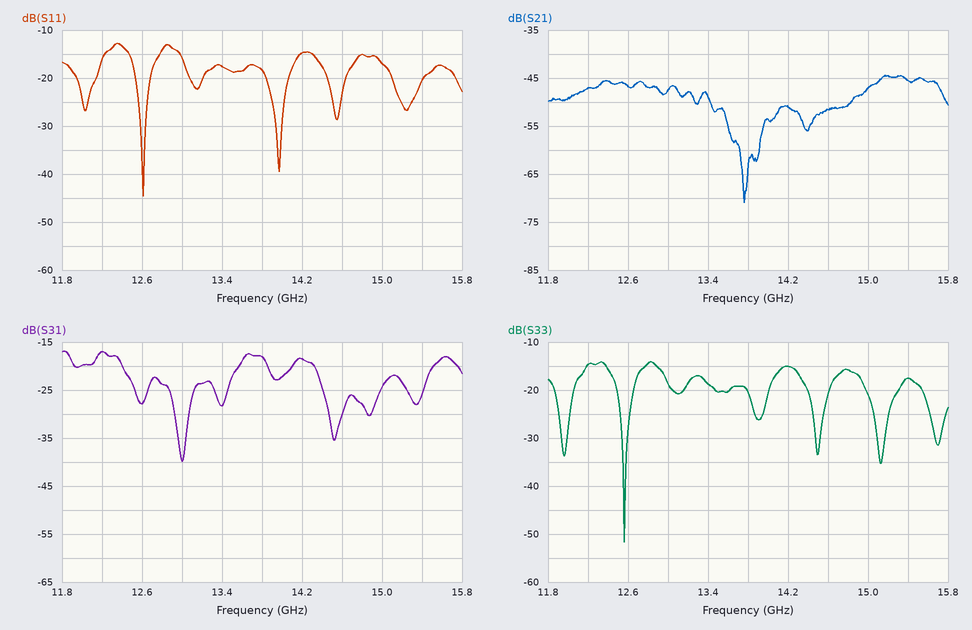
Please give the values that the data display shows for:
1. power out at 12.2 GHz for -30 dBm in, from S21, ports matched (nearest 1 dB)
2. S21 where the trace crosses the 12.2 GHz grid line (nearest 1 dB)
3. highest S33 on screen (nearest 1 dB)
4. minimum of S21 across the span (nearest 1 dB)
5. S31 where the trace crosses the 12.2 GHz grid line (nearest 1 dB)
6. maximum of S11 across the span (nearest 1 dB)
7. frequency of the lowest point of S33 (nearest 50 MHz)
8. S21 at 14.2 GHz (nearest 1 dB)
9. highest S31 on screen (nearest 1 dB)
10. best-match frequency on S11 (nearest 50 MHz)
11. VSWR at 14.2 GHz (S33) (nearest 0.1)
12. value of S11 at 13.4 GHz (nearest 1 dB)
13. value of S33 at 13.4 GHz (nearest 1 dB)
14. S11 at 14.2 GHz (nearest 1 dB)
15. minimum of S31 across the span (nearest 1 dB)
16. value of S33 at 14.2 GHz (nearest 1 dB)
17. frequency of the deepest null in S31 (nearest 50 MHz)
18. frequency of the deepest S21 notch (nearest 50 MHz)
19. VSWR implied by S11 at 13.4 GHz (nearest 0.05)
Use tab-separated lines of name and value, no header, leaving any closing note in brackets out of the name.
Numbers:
power out at 12.2 GHz for -30 dBm in, from S21, ports matched	-77 dBm
S21 where the trace crosses the 12.2 GHz grid line	-47 dB
highest S33 on screen	-14 dB
minimum of S21 across the span	-71 dB
S31 where the trace crosses the 12.2 GHz grid line	-17 dB
maximum of S11 across the span	-13 dB
frequency of the lowest point of S33	12.55 GHz
S21 at 14.2 GHz	-51 dB
highest S31 on screen	-17 dB
best-match frequency on S11	12.60 GHz
VSWR at 14.2 GHz (S33)	1.4
value of S11 at 13.4 GHz	-18 dB
value of S33 at 13.4 GHz	-19 dB
S11 at 14.2 GHz	-15 dB
minimum of S31 across the span	-40 dB
value of S33 at 14.2 GHz	-15 dB
frequency of the deepest null in S31	13.00 GHz
frequency of the deepest S21 notch	13.75 GHz
VSWR implied by S11 at 13.4 GHz	1.30
